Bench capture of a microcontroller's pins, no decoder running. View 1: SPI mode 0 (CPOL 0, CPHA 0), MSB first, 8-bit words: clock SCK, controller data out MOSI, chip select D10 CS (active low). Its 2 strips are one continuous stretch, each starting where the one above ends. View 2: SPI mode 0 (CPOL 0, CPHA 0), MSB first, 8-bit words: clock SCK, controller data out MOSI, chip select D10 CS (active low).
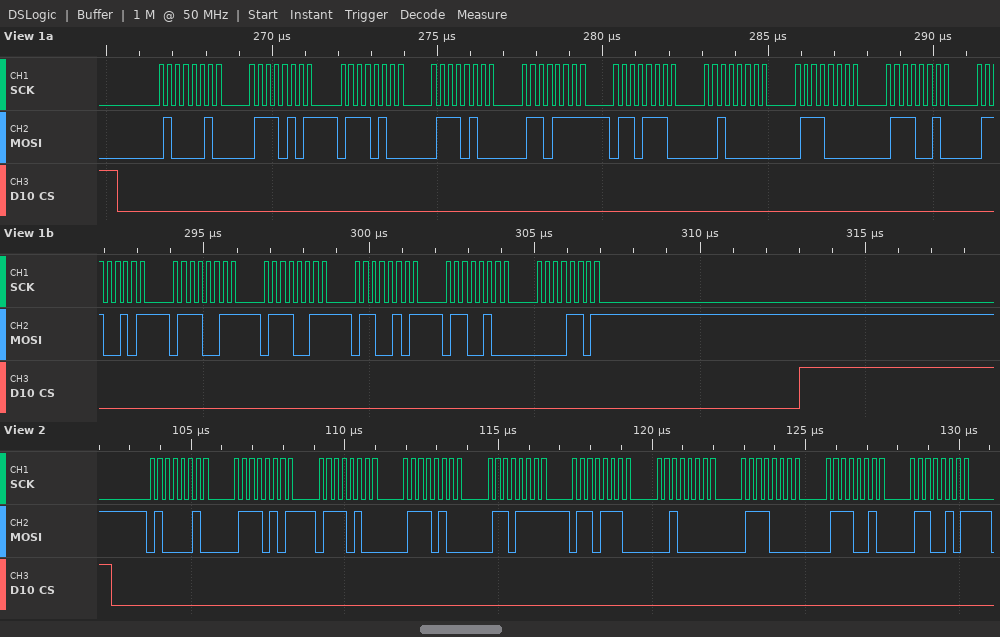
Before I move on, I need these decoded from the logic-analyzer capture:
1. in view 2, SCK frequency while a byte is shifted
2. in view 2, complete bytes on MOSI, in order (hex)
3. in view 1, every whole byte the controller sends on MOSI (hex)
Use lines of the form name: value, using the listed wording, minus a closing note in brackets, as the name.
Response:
in view 2, SCK frequency while a byte is shifted: 4 MHz
in view 2, complete bytes on MOSI, in order: 42 75 74 74 6F 6E 20 70 72 65
in view 1, every whole byte the controller sends on MOSI: 0x42 0x75 0x74 0x74 0x6F 0x6E 0x20 0x70 0x72 0x65 0x73 0x73 0x65 0x64 0x0D
